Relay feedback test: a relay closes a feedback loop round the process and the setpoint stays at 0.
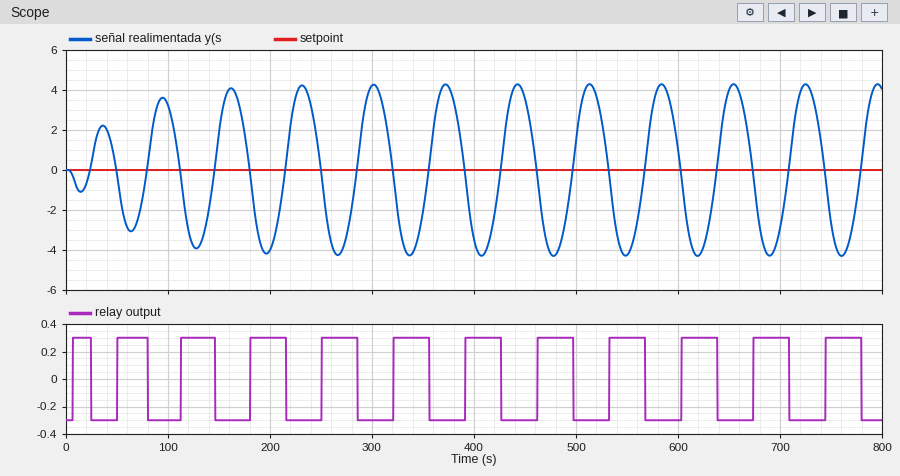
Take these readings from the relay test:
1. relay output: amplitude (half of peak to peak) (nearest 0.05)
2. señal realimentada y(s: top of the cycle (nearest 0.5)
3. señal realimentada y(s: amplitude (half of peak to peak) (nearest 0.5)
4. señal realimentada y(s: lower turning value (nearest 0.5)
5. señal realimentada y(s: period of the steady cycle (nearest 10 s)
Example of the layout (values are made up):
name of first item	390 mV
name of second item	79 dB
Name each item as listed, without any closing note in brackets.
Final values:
relay output: amplitude (half of peak to peak)	0.30
señal realimentada y(s: top of the cycle	4.5
señal realimentada y(s: amplitude (half of peak to peak)	4.5
señal realimentada y(s: lower turning value	-4.5
señal realimentada y(s: period of the steady cycle	70 s
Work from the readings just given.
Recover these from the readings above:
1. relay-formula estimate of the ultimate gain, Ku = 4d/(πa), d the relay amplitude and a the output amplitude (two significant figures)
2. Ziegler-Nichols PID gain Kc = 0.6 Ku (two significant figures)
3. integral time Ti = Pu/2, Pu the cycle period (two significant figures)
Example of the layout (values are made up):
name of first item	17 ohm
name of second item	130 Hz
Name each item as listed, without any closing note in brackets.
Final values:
relay-formula estimate of the ultimate gain, Ku = 4d/(πa), d the relay amplitude and a the output amplitude	0.085
Ziegler-Nichols PID gain Kc = 0.6 Ku	0.051
integral time Ti = Pu/2, Pu the cycle period	35 s
